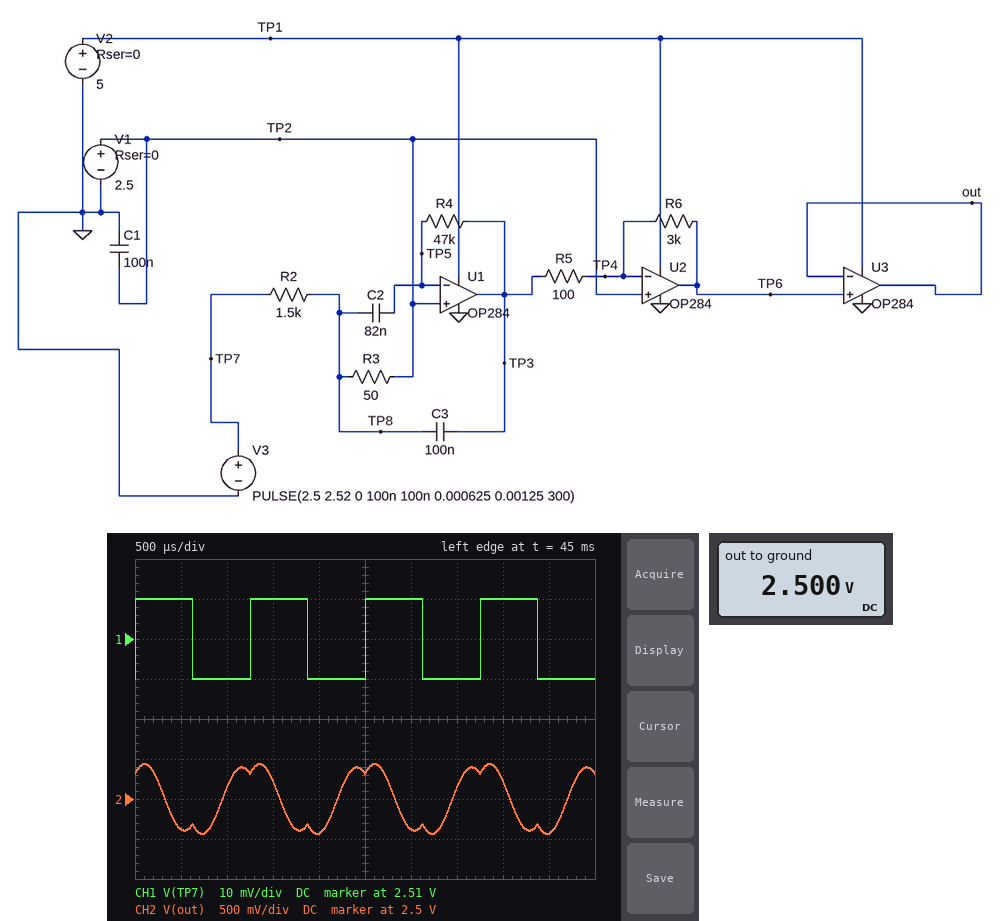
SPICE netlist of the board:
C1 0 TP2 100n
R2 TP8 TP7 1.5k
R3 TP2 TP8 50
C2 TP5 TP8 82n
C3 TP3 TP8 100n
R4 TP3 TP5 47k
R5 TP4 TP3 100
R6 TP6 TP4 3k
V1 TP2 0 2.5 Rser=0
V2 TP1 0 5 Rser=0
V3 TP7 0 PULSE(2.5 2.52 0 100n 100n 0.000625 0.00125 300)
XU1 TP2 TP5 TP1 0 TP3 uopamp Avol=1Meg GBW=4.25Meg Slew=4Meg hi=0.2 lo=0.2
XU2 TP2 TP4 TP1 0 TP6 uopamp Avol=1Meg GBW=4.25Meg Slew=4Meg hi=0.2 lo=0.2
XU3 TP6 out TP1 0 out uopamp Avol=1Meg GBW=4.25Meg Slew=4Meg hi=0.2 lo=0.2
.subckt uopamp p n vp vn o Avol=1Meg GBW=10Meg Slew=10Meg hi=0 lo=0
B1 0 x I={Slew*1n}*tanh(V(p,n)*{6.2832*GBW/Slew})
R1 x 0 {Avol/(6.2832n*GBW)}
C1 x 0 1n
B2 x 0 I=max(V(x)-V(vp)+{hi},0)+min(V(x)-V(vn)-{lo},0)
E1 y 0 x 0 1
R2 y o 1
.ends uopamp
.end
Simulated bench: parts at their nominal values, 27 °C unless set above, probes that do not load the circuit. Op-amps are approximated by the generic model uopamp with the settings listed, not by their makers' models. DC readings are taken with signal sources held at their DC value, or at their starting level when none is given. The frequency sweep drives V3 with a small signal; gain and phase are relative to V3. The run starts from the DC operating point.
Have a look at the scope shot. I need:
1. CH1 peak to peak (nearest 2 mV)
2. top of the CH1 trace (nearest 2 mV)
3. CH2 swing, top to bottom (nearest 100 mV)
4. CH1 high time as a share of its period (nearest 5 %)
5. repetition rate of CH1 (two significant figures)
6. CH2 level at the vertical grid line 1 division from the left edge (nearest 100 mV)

20 mV
2.520 V
900 mV
50 %
800 Hz
2.1 V
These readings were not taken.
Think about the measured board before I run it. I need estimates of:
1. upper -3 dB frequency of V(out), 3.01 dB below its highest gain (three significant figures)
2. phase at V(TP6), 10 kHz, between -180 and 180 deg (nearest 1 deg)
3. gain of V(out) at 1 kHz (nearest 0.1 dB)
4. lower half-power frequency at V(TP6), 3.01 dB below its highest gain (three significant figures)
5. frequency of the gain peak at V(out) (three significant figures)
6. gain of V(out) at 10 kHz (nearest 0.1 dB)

1.20 kHz
-94 deg
39.0 dB
1.12 kHz
1.16 kHz
10.1 dB
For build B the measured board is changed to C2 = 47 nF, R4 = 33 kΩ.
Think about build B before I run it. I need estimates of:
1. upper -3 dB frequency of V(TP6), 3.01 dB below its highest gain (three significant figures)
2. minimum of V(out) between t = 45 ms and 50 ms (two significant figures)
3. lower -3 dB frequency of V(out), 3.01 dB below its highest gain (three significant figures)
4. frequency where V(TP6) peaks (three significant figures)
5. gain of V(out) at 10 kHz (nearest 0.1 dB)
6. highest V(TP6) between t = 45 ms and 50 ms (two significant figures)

1.91 kHz
2.3 V
1.76 kHz
1.83 kHz
10.3 dB
2.7 V
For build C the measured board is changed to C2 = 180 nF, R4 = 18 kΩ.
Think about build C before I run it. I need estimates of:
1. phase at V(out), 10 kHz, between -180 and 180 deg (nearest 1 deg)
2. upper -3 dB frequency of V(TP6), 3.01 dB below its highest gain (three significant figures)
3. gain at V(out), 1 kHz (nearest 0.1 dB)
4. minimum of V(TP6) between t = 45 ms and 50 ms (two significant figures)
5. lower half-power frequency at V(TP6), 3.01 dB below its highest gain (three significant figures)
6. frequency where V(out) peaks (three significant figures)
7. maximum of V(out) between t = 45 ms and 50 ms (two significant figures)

-94 deg
1.34 kHz
34.2 dB
2.2 V
1.20 kHz
1.27 kHz
2.8 V
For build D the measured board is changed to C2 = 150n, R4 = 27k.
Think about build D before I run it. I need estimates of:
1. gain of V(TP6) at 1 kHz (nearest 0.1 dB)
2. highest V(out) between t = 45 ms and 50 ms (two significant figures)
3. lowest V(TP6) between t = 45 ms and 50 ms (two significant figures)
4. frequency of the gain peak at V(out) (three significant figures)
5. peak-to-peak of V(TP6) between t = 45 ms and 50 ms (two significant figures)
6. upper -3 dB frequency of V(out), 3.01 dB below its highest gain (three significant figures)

40.5 dB
3.0 V
2.0 V
1.13 kHz
970 mV
1.18 kHz
